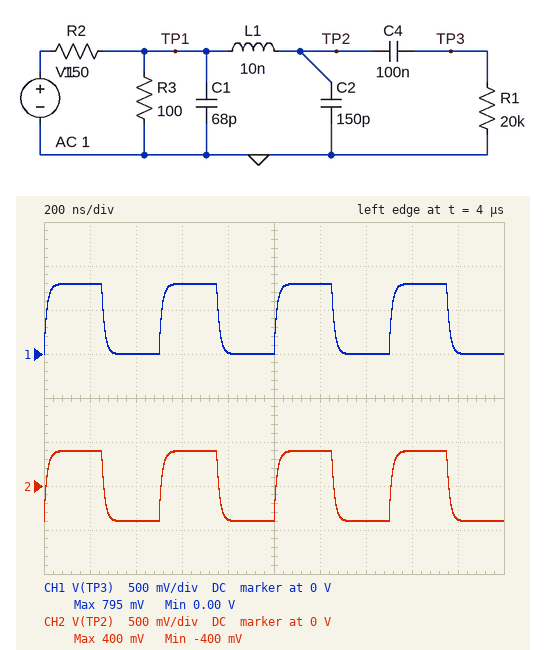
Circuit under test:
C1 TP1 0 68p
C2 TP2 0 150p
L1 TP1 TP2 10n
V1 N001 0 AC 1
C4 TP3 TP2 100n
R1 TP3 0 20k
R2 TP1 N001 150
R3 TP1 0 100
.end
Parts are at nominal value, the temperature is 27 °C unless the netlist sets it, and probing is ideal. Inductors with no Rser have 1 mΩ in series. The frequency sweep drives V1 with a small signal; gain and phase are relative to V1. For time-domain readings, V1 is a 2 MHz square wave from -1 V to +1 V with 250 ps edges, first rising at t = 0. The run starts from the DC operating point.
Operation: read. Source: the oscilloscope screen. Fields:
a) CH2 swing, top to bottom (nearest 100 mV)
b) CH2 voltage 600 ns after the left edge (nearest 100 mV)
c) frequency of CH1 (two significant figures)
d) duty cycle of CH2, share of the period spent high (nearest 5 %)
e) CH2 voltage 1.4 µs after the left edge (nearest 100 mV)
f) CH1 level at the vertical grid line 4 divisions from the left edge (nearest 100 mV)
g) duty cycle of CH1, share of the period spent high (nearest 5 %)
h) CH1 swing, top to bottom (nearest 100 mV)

800 mV
400 mV
2.0 MHz
50 %
-400 mV
0 V
50 %
800 mV
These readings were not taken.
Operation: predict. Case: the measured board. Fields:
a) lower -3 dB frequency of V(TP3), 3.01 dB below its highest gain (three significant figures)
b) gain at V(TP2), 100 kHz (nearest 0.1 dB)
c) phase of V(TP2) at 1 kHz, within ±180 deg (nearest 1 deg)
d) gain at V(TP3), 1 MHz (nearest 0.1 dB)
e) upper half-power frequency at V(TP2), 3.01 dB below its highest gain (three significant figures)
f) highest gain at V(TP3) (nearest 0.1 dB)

79.3 Hz
-8.0 dB
0 deg
-8.0 dB
12.3 MHz
-8.0 dB
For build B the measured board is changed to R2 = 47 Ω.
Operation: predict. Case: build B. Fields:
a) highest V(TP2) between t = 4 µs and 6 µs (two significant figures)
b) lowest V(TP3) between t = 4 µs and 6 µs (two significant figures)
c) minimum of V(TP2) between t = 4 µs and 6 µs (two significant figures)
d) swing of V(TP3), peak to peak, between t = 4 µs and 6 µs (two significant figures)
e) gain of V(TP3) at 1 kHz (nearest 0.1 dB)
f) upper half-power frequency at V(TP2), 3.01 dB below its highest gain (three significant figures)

680 mV
-2.0 mV
-680 mV
1.4 V
-3.4 dB
23.8 MHz
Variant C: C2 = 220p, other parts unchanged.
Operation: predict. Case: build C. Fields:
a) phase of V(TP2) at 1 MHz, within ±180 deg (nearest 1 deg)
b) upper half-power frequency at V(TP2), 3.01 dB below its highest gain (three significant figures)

-6 deg
9.27 MHz
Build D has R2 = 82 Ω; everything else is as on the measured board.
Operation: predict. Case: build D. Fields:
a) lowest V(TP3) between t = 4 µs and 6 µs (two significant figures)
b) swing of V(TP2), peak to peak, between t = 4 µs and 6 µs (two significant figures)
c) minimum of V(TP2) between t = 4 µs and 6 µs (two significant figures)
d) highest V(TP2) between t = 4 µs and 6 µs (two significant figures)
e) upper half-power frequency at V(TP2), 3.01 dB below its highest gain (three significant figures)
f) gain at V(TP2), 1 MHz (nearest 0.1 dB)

-1.6 mV
1.1 V
-550 mV
550 mV
16.5 MHz
-5.2 dB
